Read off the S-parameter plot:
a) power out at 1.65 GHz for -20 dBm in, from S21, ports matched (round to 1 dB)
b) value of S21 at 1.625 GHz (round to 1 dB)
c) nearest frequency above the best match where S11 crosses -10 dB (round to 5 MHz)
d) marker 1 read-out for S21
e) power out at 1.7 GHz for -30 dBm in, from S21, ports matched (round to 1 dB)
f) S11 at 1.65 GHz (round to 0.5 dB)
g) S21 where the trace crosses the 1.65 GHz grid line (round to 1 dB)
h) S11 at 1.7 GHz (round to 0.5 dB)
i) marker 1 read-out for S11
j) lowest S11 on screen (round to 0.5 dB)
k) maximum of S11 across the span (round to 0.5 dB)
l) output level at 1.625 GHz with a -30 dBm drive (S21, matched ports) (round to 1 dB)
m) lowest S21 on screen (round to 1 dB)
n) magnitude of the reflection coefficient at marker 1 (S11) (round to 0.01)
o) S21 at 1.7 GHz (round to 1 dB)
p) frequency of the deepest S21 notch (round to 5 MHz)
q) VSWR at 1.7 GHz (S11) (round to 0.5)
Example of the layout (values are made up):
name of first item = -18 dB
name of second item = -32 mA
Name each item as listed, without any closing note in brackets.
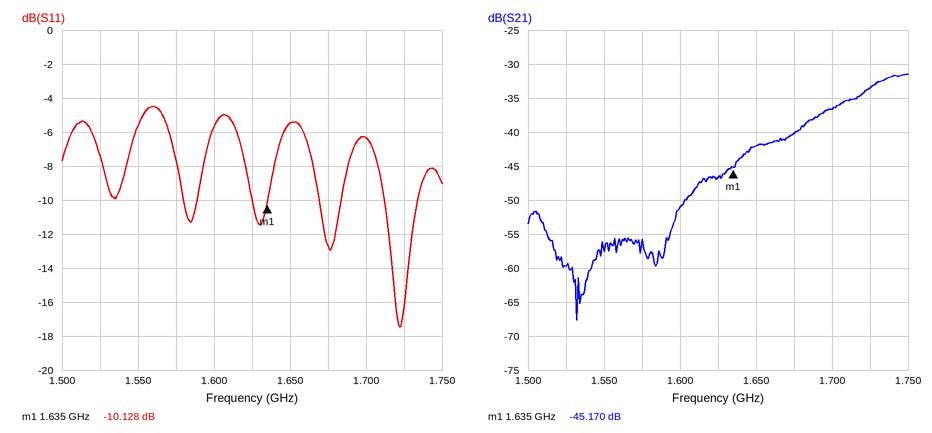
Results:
power out at 1.65 GHz for -20 dBm in, from S21, ports matched = -62 dBm
value of S21 at 1.625 GHz = -47 dB
nearest frequency above the best match where S11 crosses -10 dB = 1.735 GHz
marker 1 read-out for S21 = -45.170 dB
power out at 1.7 GHz for -30 dBm in, from S21, ports matched = -67 dBm
S11 at 1.65 GHz = -5.5 dB
S21 where the trace crosses the 1.65 GHz grid line = -42 dB
S11 at 1.7 GHz = -6.5 dB
marker 1 read-out for S11 = -10.128 dB
lowest S11 on screen = -17.5 dB
maximum of S11 across the span = -4.5 dB
output level at 1.625 GHz with a -30 dBm drive (S21, matched ports) = -77 dBm
lowest S21 on screen = -68 dB
magnitude of the reflection coefficient at marker 1 (S11) = 0.31
S21 at 1.7 GHz = -37 dB
frequency of the deepest S21 notch = 1.530 GHz
VSWR at 1.7 GHz (S11) = 3.0
